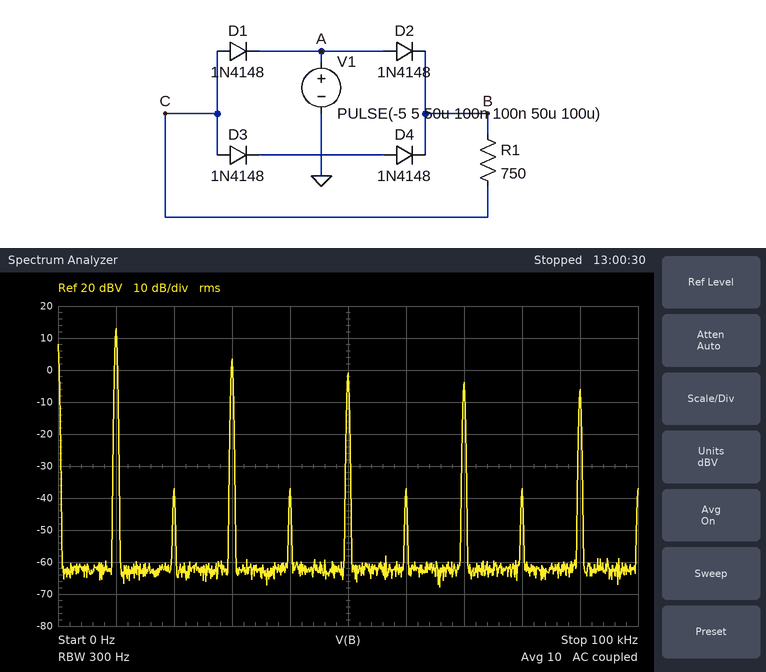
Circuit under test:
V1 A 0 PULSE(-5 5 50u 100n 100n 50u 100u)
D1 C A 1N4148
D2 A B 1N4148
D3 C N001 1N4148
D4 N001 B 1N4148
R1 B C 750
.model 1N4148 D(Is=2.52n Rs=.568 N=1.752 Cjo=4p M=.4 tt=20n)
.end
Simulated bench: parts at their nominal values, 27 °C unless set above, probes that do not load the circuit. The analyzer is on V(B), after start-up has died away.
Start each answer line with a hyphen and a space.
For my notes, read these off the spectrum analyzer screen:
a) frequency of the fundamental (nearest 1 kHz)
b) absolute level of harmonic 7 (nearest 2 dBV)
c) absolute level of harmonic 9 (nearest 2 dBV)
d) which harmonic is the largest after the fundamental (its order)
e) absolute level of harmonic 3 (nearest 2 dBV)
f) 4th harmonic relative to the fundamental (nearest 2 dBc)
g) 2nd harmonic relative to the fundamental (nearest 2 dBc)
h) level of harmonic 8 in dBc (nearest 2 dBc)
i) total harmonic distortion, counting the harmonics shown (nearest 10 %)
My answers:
- 10 kHz
- -4 dBV
- -6 dBV
- 3
- 4 dBV
- -50 dBc
- -50 dBc
- -50 dBc
- 40 %
